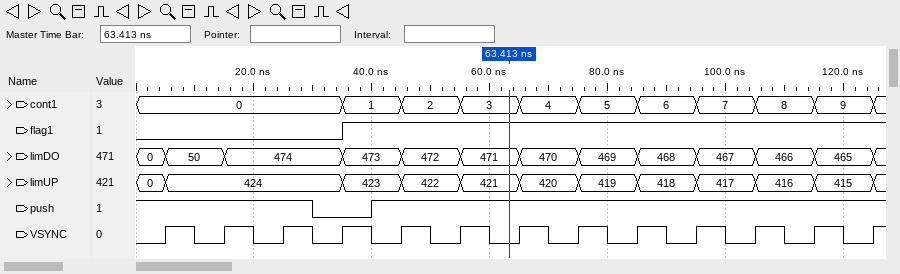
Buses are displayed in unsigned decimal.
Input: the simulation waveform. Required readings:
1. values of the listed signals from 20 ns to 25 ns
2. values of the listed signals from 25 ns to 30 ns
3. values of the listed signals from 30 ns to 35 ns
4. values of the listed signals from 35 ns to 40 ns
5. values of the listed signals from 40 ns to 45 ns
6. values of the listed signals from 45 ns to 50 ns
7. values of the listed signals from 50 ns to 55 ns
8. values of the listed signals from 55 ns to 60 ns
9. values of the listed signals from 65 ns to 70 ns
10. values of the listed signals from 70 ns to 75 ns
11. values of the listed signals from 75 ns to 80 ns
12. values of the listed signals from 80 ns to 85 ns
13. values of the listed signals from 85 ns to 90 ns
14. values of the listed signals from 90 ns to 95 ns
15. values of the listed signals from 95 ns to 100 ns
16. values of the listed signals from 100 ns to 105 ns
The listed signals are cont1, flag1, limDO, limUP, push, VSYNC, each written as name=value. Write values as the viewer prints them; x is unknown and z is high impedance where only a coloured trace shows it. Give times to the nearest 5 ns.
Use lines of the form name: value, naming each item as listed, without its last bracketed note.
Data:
values of the listed signals from 20 ns to 25 ns: cont1=0, flag1=0, limDO=474, limUP=424, push=1, VSYNC=0
values of the listed signals from 25 ns to 30 ns: cont1=0, flag1=0, limDO=474, limUP=424, push=1, VSYNC=1
values of the listed signals from 30 ns to 35 ns: cont1=0, flag1=0, limDO=474, limUP=424, push=0, VSYNC=0
values of the listed signals from 35 ns to 40 ns: cont1=1, flag1=1, limDO=473, limUP=423, push=0, VSYNC=1
values of the listed signals from 40 ns to 45 ns: cont1=1, flag1=1, limDO=473, limUP=423, push=1, VSYNC=0
values of the listed signals from 45 ns to 50 ns: cont1=2, flag1=1, limDO=472, limUP=422, push=1, VSYNC=1
values of the listed signals from 50 ns to 55 ns: cont1=2, flag1=1, limDO=472, limUP=422, push=1, VSYNC=0
values of the listed signals from 55 ns to 60 ns: cont1=3, flag1=1, limDO=471, limUP=421, push=1, VSYNC=1
values of the listed signals from 65 ns to 70 ns: cont1=4, flag1=1, limDO=470, limUP=420, push=1, VSYNC=1
values of the listed signals from 70 ns to 75 ns: cont1=4, flag1=1, limDO=470, limUP=420, push=1, VSYNC=0
values of the listed signals from 75 ns to 80 ns: cont1=5, flag1=1, limDO=469, limUP=419, push=1, VSYNC=1
values of the listed signals from 80 ns to 85 ns: cont1=5, flag1=1, limDO=469, limUP=419, push=1, VSYNC=0
values of the listed signals from 85 ns to 90 ns: cont1=6, flag1=1, limDO=468, limUP=418, push=1, VSYNC=1
values of the listed signals from 90 ns to 95 ns: cont1=6, flag1=1, limDO=468, limUP=418, push=1, VSYNC=0
values of the listed signals from 95 ns to 100 ns: cont1=7, flag1=1, limDO=467, limUP=417, push=1, VSYNC=1
values of the listed signals from 100 ns to 105 ns: cont1=7, flag1=1, limDO=467, limUP=417, push=1, VSYNC=0
